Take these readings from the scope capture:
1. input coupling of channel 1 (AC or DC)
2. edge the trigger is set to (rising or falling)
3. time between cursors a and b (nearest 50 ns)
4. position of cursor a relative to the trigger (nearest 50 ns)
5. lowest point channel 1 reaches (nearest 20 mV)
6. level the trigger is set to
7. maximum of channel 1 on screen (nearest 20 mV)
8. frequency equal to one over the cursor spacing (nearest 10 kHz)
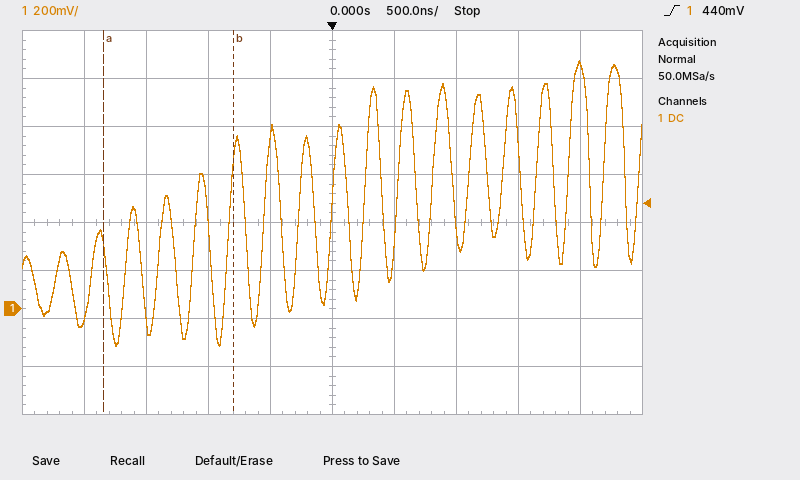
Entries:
DC
rising
1.05 µs
-1.85 µs
-160 mV
440 mV
1.04 V
950 kHz
